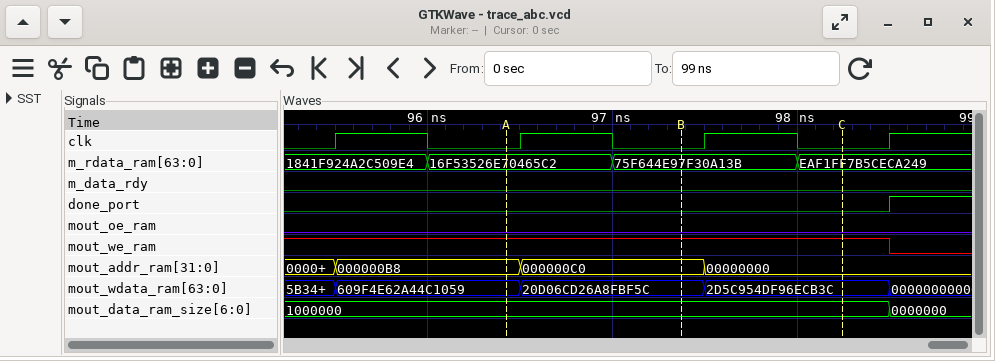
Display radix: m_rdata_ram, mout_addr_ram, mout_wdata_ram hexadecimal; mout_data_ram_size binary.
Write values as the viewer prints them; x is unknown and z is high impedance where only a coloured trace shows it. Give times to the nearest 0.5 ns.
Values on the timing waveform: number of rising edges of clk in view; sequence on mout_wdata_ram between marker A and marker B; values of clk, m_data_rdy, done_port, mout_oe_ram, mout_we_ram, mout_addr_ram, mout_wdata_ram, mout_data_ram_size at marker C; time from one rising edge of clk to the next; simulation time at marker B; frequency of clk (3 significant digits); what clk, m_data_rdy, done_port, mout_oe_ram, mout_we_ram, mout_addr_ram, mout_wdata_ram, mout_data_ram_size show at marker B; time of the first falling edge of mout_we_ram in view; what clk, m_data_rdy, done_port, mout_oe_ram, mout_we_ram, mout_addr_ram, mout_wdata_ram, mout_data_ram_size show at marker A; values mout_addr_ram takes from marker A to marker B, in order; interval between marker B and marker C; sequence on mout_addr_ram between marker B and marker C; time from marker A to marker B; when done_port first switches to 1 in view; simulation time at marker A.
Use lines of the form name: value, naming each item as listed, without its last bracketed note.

number of rising edges of clk in view: 4
sequence on mout_wdata_ram between marker A and marker B: 609F4E62A44C1059, 20D06CD26A8FBF5C
values of clk, m_data_rdy, done_port, mout_oe_ram, mout_we_ram, mout_addr_ram, mout_wdata_ram, mout_data_ram_size at marker C: clk=0, m_data_rdy=0, done_port=0, mout_oe_ram=0, mout_we_ram=1, mout_addr_ram=00000000, mout_wdata_ram=2D5C954DF96ECB3C, mout_data_ram_size=1000000
time from one rising edge of clk to the next: 1 ns
simulation time at marker B: 97.5 ns
frequency of clk: 1.00 GHz
what clk, m_data_rdy, done_port, mout_oe_ram, mout_we_ram, mout_addr_ram, mout_wdata_ram, mout_data_ram_size show at marker B: clk=0, m_data_rdy=0, done_port=0, mout_oe_ram=0, mout_we_ram=1, mout_addr_ram=000000C0, mout_wdata_ram=20D06CD26A8FBF5C, mout_data_ram_size=1000000
time of the first falling edge of mout_we_ram in view: 98.5 ns
what clk, m_data_rdy, done_port, mout_oe_ram, mout_we_ram, mout_addr_ram, mout_wdata_ram, mout_data_ram_size show at marker A: clk=0, m_data_rdy=0, done_port=0, mout_oe_ram=0, mout_we_ram=1, mout_addr_ram=000000B8, mout_wdata_ram=609F4E62A44C1059, mout_data_ram_size=1000000
values mout_addr_ram takes from marker A to marker B, in order: 000000B8, 000000C0
interval between marker B and marker C: 1 ns
sequence on mout_addr_ram between marker B and marker C: 000000C0, 00000000
time from marker A to marker B: 1 ns
when done_port first switches to 1 in view: 98.5 ns
simulation time at marker A: 96.5 ns
